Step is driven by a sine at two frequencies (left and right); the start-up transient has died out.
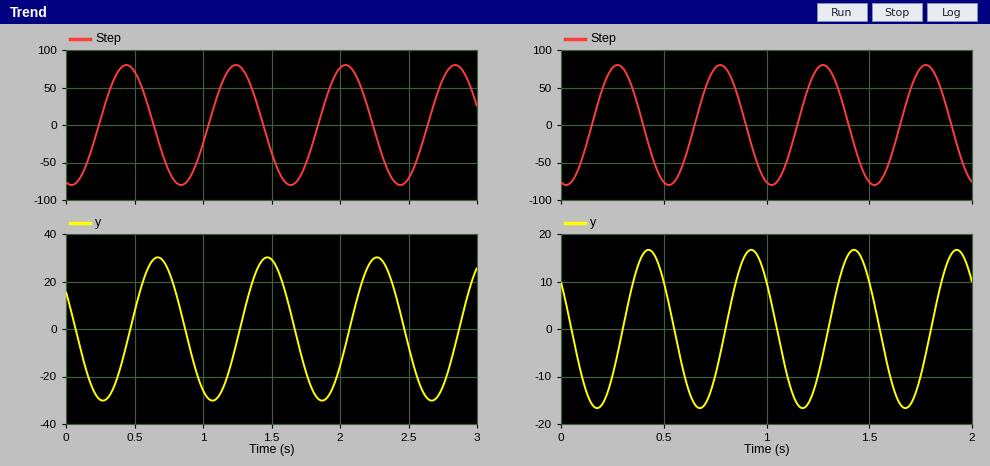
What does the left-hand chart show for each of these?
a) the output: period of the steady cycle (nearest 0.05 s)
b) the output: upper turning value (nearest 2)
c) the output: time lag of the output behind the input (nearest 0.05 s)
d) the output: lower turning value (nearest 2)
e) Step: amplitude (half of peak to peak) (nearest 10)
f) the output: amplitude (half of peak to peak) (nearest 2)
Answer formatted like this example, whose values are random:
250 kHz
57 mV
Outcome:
0.80 s
30
0.25 s
-30
80
30
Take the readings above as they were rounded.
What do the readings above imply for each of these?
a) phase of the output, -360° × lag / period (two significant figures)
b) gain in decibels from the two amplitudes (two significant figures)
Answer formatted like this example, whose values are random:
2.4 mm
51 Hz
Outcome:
-110°
-8.5 dB
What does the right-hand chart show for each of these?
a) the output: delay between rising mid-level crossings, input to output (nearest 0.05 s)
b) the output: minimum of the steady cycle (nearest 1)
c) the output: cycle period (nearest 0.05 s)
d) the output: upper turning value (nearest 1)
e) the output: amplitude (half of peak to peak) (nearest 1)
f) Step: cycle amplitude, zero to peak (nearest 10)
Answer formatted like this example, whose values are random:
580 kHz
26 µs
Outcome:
0.15 s
-17
0.50 s
17
17
80
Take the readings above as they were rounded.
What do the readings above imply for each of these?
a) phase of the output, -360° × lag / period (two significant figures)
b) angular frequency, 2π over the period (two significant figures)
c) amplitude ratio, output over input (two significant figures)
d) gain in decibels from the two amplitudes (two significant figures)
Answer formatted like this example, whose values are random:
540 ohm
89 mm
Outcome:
-110°
13 rad/s
0.21
-13 dB
